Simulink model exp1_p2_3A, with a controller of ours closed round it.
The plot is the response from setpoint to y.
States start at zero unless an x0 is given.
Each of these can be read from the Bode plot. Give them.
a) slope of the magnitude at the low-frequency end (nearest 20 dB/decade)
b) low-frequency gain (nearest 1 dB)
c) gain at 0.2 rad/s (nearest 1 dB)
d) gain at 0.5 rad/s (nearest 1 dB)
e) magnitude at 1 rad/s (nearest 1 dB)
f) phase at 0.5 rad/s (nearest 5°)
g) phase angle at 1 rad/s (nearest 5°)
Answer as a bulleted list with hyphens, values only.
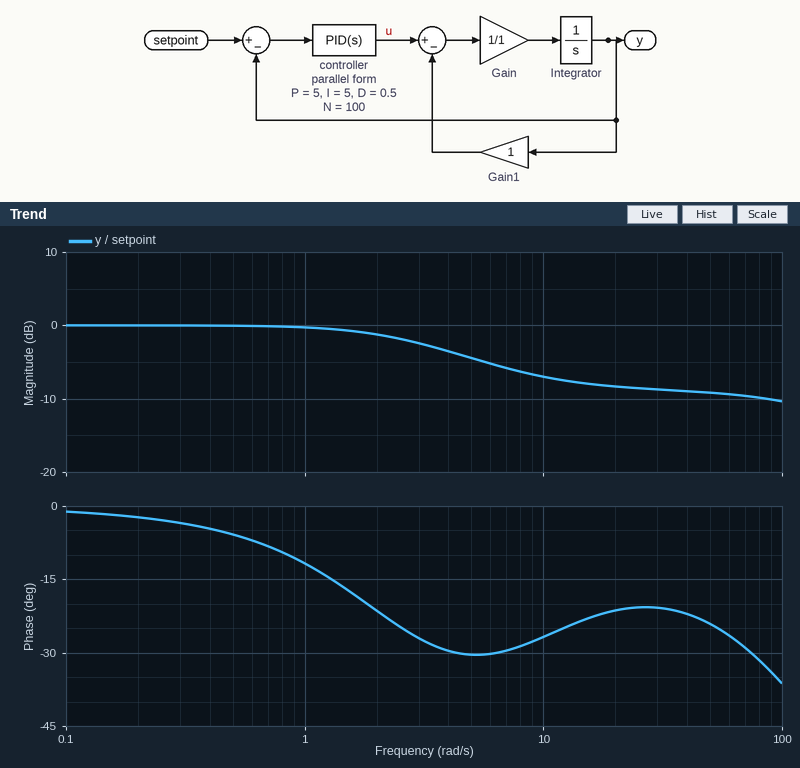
- 0 dB/decade
- 0 dB
- 0 dB
- 0 dB
- 0 dB
- -5°
- -10°
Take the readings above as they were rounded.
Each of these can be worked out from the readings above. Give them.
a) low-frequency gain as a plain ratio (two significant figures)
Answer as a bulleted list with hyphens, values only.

- 1.0
